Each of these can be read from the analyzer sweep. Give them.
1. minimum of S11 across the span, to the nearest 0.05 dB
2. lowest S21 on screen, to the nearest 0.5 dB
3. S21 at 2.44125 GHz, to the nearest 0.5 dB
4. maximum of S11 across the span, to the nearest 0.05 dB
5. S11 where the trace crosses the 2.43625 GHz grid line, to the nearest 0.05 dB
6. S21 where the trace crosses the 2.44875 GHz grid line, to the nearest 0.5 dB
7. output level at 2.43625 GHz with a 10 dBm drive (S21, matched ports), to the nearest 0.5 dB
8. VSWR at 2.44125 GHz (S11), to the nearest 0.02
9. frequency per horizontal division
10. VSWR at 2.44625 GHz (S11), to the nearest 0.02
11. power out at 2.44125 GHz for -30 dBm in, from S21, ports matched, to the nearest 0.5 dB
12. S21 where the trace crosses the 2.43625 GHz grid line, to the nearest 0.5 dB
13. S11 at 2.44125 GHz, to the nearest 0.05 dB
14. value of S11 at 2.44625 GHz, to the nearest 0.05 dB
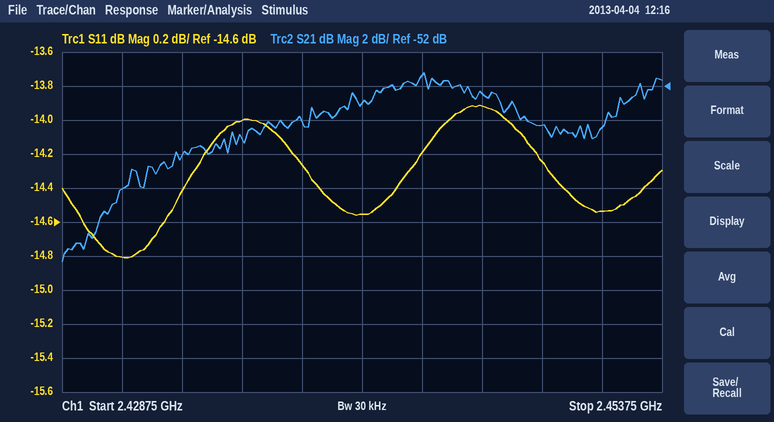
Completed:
-14.80 dB
-62.5 dB
-53.0 dB
-13.90 dB
-14.00 dB
-54.5 dB
-45.0 dBm
1.46
2.5 MHz
1.50
-83.0 dBm
-55.0 dB
-14.55 dB
-13.90 dB
